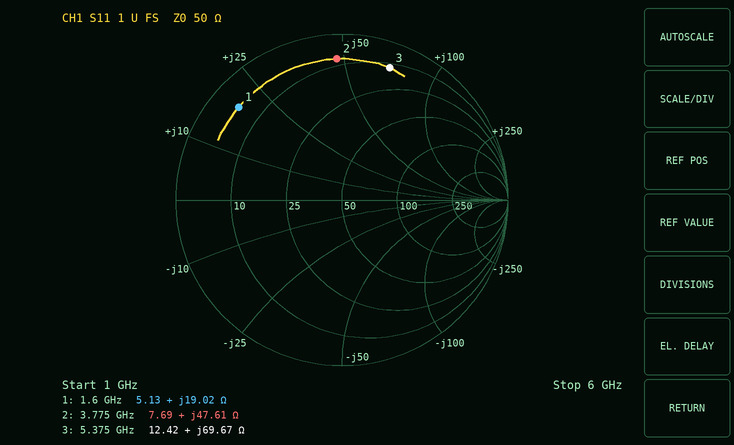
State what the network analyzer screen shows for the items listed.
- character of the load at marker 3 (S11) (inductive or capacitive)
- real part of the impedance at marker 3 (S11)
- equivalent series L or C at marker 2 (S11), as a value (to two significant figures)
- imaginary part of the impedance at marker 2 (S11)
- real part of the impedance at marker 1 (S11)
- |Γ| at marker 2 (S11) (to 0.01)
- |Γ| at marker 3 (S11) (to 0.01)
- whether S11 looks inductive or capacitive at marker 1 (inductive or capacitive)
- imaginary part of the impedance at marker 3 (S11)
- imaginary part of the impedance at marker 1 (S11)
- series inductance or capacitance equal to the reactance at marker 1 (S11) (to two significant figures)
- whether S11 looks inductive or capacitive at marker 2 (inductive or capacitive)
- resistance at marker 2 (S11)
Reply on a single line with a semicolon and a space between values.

inductive; 12.42 Ω; 2.0 nH; +47.61 Ω; 5.13 Ω; 0.85; 0.85; inductive; +69.67 Ω; +19.02 Ω; 1.9 nH; inductive; 7.69 Ω
